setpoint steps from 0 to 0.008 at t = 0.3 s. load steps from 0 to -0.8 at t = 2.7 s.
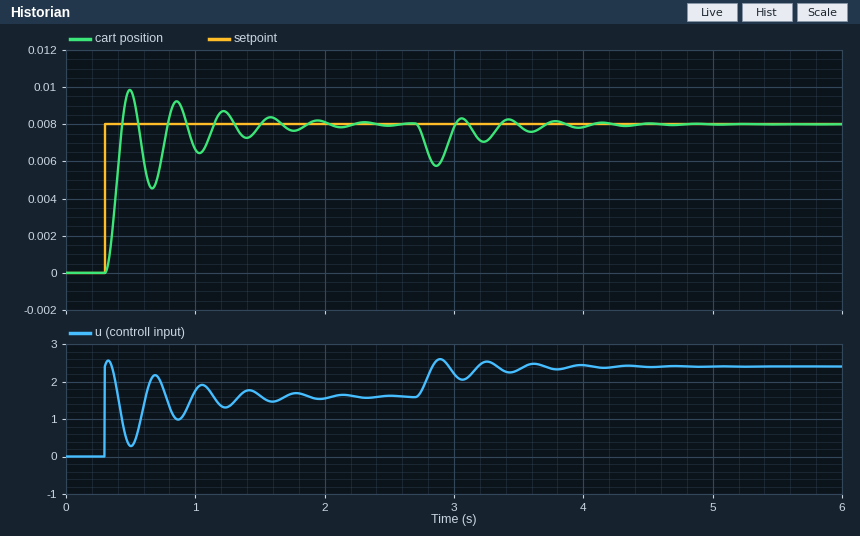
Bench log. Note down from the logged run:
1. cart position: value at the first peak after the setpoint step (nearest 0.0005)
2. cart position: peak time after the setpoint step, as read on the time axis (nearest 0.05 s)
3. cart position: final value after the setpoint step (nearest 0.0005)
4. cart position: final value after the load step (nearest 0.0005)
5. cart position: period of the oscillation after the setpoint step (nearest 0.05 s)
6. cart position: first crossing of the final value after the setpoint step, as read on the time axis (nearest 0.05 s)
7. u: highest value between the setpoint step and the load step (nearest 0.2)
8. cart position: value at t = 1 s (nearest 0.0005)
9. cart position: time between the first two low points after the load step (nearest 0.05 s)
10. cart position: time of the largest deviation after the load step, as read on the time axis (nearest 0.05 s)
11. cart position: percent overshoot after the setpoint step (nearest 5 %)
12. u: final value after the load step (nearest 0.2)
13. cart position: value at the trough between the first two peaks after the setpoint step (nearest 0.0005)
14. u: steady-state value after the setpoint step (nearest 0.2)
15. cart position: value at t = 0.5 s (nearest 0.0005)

0.0100
0.50 s
0.0080
0.0080
0.35 s
0.45 s
2.6
0.0065
0.35 s
2.85 s
25 %
2.4
0.0045
1.6
0.0100
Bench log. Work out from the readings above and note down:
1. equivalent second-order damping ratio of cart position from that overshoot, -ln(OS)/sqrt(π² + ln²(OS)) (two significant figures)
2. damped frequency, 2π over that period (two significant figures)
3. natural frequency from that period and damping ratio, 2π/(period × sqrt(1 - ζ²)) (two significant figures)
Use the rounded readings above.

0.40
18 rad/s
20 rad/s
